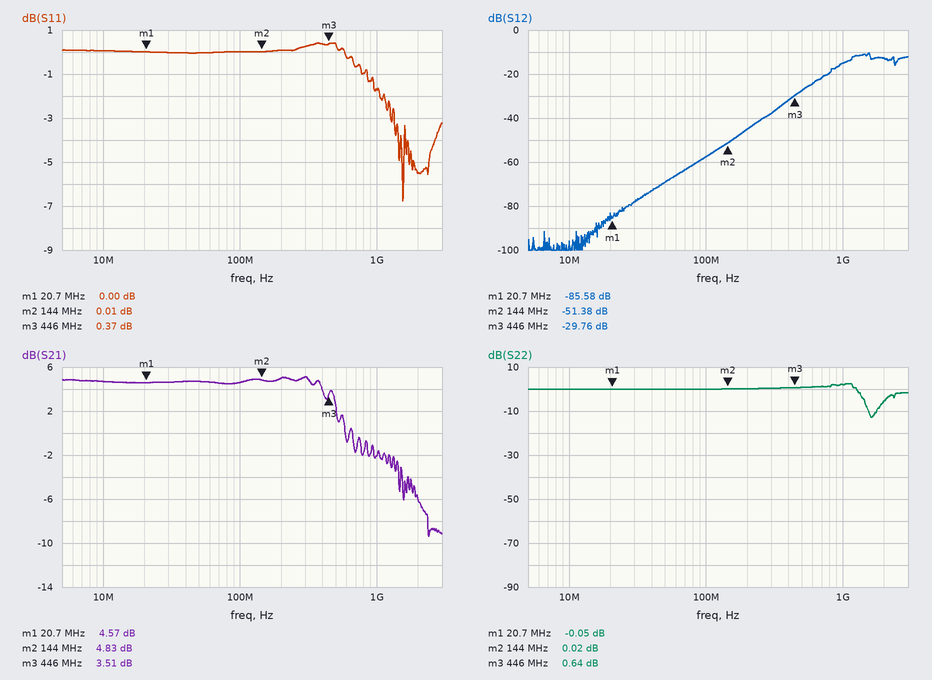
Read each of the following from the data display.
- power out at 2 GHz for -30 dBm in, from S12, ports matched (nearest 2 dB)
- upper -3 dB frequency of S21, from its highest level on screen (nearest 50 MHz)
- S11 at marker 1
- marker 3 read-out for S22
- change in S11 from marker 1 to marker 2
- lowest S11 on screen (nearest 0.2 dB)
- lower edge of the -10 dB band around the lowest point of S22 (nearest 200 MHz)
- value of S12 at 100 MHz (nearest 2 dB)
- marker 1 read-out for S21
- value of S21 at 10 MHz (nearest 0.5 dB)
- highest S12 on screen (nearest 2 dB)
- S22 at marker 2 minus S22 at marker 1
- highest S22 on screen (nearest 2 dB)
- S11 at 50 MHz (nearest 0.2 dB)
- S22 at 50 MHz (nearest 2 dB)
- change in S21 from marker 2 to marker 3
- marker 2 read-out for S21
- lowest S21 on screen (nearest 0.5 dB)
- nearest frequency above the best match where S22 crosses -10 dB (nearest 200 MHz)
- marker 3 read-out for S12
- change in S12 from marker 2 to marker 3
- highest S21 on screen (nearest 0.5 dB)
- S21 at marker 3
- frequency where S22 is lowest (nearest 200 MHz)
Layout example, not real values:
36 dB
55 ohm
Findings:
-42 dBm
500 MHz
0.00 dB
0.64 dB
0.01 dB
-6.8 dB
1.6 GHz
-58 dB
4.57 dB
4.5 dB
-10 dB
0.07 dB
2 dB
0.0 dB
0 dB
-1.32 dB
4.83 dB
-9.5 dB
1.8 GHz
-29.76 dB
21.62 dB
5.0 dB
3.51 dB
1.6 GHz
